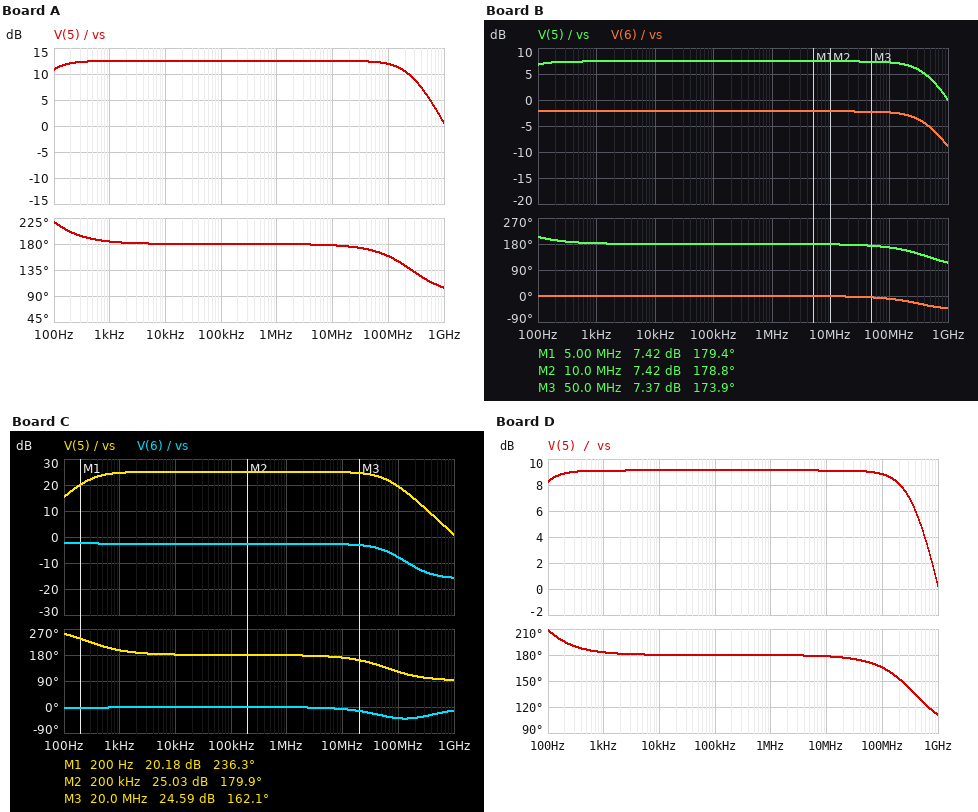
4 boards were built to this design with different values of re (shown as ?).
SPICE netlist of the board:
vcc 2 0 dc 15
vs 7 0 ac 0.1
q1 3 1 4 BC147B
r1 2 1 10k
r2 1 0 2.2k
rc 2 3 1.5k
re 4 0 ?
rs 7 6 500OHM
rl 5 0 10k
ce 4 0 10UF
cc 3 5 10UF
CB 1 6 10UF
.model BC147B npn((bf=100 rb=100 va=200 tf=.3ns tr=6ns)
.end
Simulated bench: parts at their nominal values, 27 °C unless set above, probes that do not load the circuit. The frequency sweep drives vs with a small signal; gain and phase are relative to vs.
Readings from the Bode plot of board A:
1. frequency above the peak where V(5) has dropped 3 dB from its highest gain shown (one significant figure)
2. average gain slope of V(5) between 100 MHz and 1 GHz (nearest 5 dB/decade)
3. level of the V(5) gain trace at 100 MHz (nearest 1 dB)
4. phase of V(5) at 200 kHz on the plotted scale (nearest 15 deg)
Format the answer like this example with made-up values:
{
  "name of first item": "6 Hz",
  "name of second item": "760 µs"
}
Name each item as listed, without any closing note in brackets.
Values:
{
  "frequency above the peak where V(5) has dropped 3 dB from its highest gain shown": "300 MHz",
  "average gain slope of V(5) between 100 MHz and 1 GHz": "-10 dB/decade",
  "level of the V(5) gain trace at 100 MHz": "12 dB",
  "phase of V(5) at 200 kHz on the plotted scale": "180 deg"
}
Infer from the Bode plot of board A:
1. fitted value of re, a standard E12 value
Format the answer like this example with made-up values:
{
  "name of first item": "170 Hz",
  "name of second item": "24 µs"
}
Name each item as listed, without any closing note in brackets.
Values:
{
  "fitted value of re, a standard E12 value": "18 kΩ"
}
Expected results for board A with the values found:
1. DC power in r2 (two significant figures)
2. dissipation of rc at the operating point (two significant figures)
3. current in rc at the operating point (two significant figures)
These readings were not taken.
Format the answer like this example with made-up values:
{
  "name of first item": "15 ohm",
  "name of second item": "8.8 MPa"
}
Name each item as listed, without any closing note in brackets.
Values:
{
  "DC power in r2": "3.3 mW",
  "dissipation of rc at the operating point": "18 µW",
  "current in rc at the operating point": "110 µA"
}
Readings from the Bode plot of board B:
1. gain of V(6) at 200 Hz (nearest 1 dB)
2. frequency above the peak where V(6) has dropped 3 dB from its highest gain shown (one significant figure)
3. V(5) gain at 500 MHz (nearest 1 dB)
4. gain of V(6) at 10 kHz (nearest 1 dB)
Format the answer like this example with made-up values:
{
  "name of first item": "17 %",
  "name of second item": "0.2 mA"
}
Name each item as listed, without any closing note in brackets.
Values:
{
  "gain of V(6) at 200 Hz": "-2 dB",
  "frequency above the peak where V(6) has dropped 3 dB from its highest gain shown": "500 MHz",
  "V(5) gain at 500 MHz": "4 dB",
  "gain of V(6) at 10 kHz": "-2 dB"
}
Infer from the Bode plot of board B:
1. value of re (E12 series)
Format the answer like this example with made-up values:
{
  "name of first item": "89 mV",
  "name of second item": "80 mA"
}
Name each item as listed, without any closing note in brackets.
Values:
{
  "value of re": "33 kΩ"
}
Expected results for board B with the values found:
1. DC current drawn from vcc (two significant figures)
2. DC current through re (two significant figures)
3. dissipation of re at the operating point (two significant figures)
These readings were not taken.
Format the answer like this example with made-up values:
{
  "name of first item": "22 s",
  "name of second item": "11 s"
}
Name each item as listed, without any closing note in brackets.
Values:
{
  "DC current drawn from vcc": "1.3 mA",
  "DC current through re": "61 µA",
  "dissipation of re at the operating point": "120 µW"
}
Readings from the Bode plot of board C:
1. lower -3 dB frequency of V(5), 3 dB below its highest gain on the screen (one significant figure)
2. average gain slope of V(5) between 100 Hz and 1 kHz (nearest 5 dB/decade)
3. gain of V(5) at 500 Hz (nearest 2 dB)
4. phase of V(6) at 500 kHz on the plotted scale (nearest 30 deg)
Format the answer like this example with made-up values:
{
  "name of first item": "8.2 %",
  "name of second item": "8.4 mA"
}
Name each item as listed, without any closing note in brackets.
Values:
{
  "lower -3 dB frequency of V(5), 3 dB below its highest gain on the screen": "300 Hz",
  "average gain slope of V(5) between 100 Hz and 1 kHz": "10 dB/decade",
  "gain of V(5) at 500 Hz": "24 dB",
  "phase of V(6) at 500 kHz on the plotted scale": "0 deg"
}
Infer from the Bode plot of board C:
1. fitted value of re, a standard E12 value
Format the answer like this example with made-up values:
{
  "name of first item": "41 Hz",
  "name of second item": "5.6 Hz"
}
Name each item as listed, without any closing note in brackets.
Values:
{
  "fitted value of re, a standard E12 value": "3.9 kΩ"
}
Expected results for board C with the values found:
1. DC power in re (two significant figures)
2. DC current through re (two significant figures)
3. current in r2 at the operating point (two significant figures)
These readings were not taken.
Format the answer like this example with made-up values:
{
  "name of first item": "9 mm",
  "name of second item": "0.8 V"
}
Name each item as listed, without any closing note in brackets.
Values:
{
  "DC power in re": "970 µW",
  "DC current through re": "500 µA",
  "current in r2 at the operating point": "1.2 mA"
}
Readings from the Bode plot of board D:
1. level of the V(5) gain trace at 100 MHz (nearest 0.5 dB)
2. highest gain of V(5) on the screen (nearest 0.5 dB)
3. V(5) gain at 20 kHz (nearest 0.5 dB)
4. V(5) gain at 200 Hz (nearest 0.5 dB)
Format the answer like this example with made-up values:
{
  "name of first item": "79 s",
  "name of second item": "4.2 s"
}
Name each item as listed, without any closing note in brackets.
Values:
{
  "level of the V(5) gain trace at 100 MHz": "9.0 dB",
  "highest gain of V(5) on the screen": "9.0 dB",
  "V(5) gain at 20 kHz": "9.0 dB",
  "V(5) gain at 200 Hz": "9.0 dB"
}
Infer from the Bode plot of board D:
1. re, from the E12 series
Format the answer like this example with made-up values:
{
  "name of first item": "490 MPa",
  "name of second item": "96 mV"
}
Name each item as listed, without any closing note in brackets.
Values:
{
  "re, from the E12 series": "27 kΩ"
}
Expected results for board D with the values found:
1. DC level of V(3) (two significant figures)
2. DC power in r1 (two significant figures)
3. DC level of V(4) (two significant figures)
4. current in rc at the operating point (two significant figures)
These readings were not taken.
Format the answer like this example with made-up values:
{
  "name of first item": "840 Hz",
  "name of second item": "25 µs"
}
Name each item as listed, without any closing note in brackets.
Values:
{
  "DC level of V(3)": "15 V",
  "DC power in r1": "15 mW",
  "DC level of V(4)": "2.0 V",
  "current in rc at the operating point": "73 µA"
}
